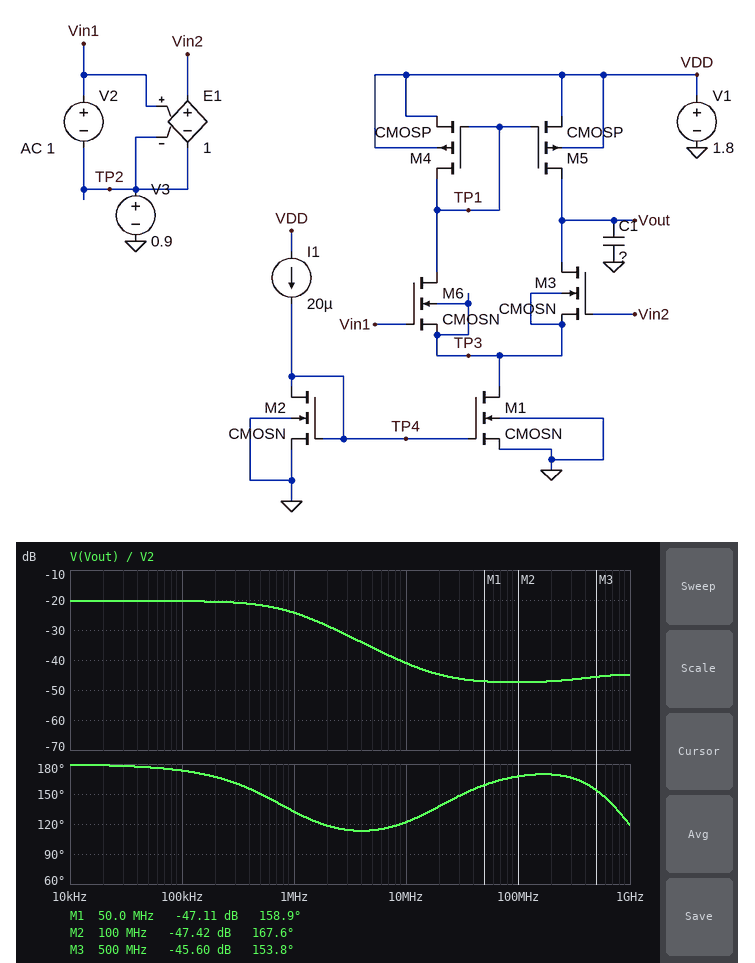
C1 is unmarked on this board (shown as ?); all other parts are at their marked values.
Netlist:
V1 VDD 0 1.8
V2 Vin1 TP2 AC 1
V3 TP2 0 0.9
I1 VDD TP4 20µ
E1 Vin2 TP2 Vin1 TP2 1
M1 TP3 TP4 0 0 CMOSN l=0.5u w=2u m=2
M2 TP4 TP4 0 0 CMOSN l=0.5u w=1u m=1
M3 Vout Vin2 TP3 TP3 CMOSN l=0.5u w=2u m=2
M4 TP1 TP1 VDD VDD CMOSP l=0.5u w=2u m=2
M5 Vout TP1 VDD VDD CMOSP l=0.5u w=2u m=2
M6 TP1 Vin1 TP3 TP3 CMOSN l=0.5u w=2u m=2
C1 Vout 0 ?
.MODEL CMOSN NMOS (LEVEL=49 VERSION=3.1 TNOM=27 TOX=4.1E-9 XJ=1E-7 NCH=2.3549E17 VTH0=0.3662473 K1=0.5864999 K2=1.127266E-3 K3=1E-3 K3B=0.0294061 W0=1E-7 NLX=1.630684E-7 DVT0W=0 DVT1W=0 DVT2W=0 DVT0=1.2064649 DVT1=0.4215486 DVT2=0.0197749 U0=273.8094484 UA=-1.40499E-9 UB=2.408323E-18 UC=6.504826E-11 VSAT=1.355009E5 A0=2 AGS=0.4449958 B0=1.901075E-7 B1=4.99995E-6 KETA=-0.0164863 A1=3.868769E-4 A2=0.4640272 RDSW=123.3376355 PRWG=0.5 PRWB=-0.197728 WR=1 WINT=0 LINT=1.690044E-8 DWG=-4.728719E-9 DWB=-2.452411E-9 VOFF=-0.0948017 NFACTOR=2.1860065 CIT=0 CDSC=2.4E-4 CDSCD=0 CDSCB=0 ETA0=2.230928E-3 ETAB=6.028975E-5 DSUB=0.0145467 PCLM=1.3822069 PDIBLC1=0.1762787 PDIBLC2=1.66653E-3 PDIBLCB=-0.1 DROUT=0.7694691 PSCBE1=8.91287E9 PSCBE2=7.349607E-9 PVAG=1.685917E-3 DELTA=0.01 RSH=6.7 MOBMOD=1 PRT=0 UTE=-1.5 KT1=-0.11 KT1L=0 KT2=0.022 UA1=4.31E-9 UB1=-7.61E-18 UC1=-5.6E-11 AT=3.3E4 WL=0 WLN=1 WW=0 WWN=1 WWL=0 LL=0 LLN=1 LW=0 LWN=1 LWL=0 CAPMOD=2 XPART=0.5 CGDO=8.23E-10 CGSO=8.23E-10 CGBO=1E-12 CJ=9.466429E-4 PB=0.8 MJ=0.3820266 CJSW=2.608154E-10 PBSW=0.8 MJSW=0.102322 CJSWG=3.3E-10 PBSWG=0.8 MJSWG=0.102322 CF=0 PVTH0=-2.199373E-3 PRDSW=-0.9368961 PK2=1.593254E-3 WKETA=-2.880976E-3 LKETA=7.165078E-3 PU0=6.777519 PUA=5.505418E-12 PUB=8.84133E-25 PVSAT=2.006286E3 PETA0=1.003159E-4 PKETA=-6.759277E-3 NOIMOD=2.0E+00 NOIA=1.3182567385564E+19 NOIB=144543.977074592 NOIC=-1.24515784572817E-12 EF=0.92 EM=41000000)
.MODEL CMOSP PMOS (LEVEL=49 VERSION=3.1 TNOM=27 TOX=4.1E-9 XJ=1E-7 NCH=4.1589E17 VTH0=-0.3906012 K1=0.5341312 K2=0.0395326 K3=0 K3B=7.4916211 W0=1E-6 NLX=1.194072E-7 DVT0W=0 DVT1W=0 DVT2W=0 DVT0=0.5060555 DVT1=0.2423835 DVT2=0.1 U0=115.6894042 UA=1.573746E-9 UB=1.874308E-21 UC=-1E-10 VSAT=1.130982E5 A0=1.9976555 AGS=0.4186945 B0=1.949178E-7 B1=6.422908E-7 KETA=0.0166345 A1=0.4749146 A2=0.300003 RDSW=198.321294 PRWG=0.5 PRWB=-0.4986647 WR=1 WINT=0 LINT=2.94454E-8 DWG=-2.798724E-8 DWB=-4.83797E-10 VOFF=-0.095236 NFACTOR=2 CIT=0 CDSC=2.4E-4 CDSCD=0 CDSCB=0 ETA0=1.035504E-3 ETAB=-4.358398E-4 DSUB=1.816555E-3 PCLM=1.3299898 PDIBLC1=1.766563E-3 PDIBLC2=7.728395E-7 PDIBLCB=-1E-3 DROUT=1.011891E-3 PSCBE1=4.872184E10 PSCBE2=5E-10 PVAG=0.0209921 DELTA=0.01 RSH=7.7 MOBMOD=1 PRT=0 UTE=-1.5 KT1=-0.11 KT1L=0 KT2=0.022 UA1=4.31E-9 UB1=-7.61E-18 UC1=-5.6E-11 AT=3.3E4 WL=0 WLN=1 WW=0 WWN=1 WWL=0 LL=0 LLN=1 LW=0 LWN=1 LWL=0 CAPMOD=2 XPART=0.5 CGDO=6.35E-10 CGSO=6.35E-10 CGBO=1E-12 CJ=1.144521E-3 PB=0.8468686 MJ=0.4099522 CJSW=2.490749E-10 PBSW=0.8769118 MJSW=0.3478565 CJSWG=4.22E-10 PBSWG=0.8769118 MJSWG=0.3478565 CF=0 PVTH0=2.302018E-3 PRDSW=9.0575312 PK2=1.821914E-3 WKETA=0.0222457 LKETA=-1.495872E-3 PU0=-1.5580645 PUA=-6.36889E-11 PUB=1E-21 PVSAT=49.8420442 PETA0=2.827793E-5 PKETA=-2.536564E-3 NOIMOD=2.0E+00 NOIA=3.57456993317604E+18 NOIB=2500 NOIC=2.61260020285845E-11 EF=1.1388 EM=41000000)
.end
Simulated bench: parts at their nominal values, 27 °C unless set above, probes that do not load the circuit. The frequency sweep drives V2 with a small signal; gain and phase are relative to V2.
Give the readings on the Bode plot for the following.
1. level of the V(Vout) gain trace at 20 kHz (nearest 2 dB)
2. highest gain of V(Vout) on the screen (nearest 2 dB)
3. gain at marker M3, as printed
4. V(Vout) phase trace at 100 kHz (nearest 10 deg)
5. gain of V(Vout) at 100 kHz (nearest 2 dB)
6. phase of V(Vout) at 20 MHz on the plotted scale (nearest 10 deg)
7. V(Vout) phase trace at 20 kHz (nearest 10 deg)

-20 dB
-20 dB
-45.60 dB
170 deg
-20 dB
140 deg
180 deg
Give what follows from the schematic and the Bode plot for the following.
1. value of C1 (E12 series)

1.2 pF
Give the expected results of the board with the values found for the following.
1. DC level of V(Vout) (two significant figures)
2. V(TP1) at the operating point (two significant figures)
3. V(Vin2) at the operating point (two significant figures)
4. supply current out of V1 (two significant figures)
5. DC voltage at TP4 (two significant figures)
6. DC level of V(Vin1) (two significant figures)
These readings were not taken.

980 mV
980 mV
900 mV
91 µA
720 mV
900 mV
